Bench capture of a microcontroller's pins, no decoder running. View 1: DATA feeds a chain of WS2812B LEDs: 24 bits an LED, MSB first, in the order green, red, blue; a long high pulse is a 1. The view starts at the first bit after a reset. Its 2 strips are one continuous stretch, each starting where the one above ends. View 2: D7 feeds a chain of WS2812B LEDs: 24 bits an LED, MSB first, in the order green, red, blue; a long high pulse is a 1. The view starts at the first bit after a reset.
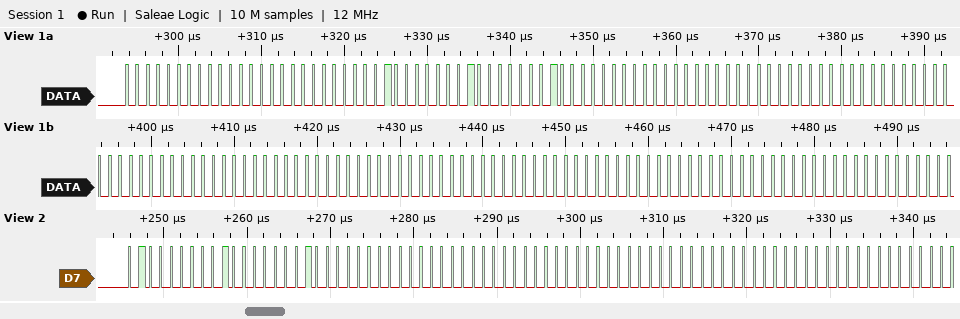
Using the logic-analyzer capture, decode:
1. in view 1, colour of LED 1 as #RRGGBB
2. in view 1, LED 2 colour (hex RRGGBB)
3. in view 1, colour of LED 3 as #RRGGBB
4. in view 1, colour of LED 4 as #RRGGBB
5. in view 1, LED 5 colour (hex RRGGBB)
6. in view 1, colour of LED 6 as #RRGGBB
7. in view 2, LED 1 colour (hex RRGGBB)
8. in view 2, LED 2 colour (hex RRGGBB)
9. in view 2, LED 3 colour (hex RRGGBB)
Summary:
#000000
#404040
#000000
#000000
#000000
#000000
#404040
#000000
#000000
